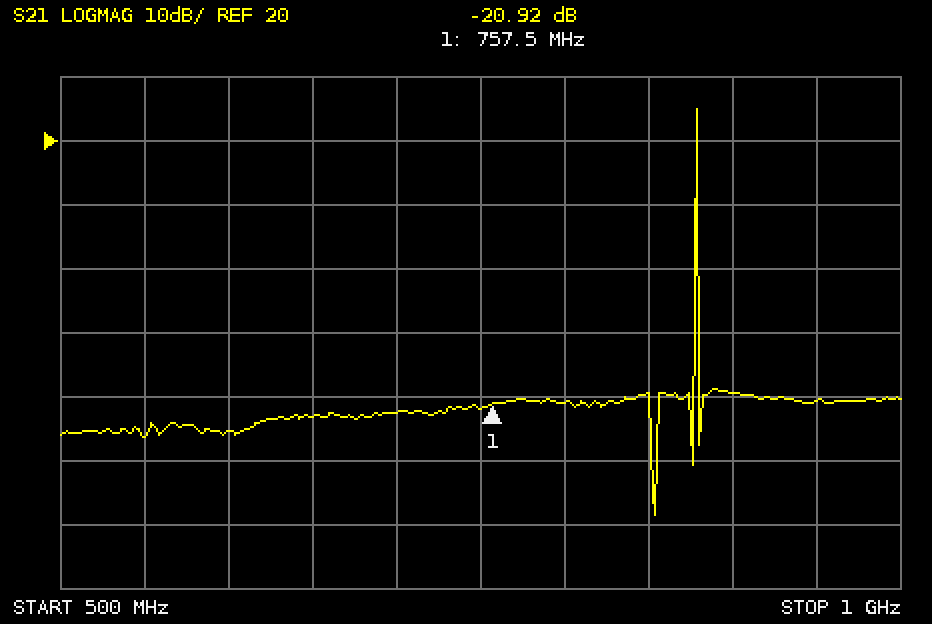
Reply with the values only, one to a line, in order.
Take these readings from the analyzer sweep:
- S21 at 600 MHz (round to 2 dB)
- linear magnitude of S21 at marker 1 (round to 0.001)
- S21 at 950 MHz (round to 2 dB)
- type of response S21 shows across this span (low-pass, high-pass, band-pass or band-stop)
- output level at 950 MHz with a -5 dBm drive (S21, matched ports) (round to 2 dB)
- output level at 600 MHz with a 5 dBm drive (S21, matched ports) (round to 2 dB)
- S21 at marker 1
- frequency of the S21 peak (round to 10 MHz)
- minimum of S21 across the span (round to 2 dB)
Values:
-26 dB
0.090
-20 dB
band-pass
-26 dBm
-20 dBm
-20.92 dB
880 MHz
-38 dB
